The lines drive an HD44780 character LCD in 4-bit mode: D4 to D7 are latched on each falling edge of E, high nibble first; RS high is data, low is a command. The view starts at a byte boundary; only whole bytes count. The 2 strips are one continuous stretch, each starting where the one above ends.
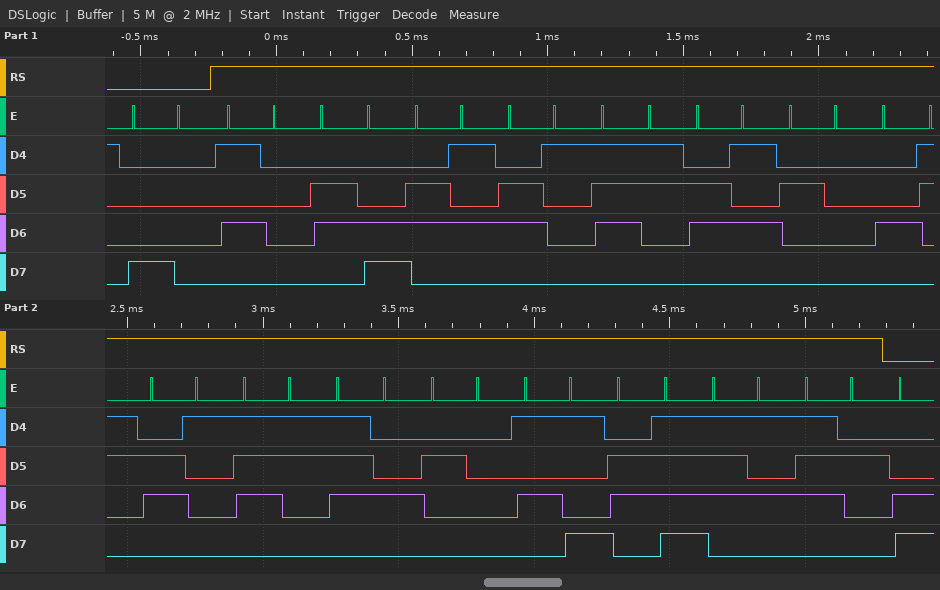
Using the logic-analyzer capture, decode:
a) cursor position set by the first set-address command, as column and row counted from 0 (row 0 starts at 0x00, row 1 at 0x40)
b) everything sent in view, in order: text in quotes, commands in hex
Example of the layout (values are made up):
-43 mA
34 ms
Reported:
column 0, row 0
0x80 "Please Cast Your"
